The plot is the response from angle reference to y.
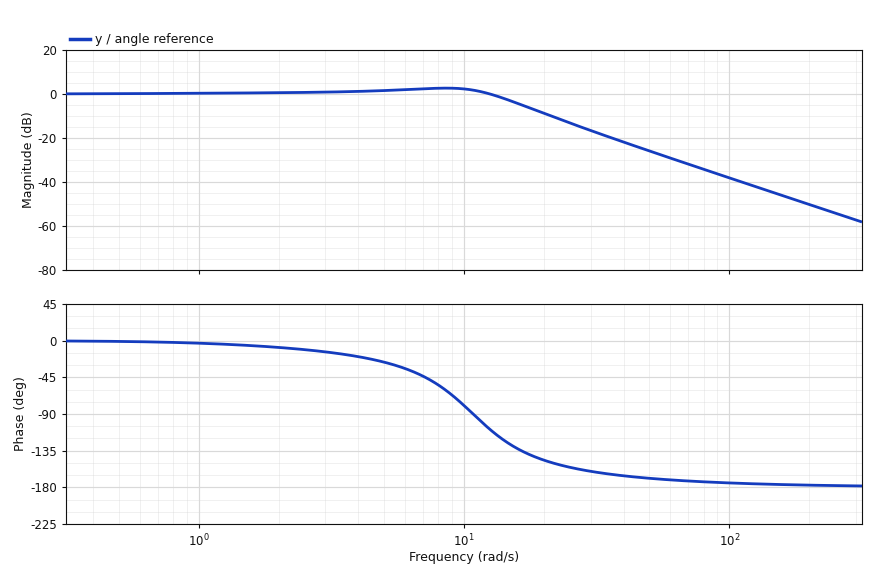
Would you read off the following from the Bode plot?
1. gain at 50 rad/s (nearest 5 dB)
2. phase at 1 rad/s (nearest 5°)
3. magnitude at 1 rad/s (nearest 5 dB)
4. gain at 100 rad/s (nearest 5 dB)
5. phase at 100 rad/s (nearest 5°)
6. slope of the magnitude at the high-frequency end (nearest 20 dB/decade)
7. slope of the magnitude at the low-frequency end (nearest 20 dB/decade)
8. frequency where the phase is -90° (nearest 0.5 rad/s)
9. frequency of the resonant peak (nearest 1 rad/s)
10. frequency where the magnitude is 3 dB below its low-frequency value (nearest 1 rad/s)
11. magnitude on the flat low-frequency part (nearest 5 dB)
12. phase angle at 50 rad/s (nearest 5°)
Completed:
-25 dB
-5°
0 dB
-40 dB
-175°
-40 dB/decade
0 dB/decade
11.0 rad/s
8 rad/s
15 rad/s
0 dB
-170°
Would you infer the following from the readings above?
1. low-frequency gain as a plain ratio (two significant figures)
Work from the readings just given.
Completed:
1.0
